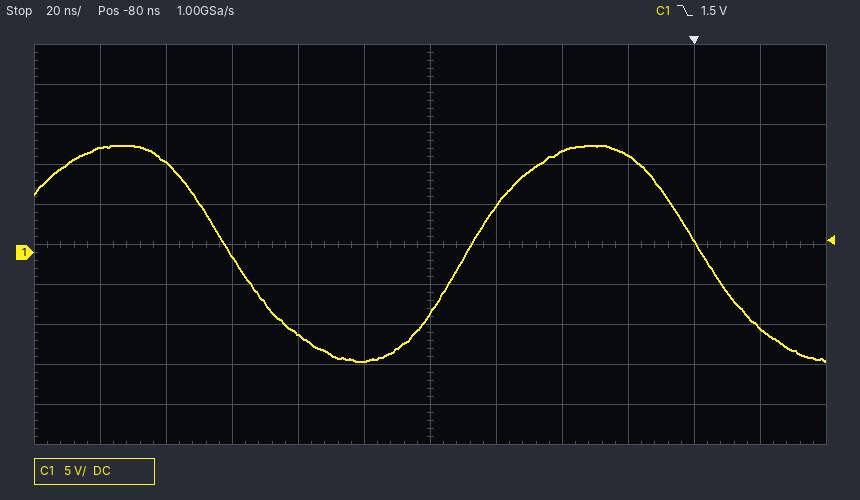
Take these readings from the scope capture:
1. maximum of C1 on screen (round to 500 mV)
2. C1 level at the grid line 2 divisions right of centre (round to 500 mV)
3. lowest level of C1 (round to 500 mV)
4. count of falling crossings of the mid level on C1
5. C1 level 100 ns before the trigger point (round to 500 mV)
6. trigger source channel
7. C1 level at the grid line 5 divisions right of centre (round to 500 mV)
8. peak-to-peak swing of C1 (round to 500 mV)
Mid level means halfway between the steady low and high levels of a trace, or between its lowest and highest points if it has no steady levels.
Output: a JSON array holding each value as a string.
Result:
["13.5 V", "12.5 V", "-13.5 V", "2", "-13.5 V", "C1", "-9.5 V", "27.0 V"]
